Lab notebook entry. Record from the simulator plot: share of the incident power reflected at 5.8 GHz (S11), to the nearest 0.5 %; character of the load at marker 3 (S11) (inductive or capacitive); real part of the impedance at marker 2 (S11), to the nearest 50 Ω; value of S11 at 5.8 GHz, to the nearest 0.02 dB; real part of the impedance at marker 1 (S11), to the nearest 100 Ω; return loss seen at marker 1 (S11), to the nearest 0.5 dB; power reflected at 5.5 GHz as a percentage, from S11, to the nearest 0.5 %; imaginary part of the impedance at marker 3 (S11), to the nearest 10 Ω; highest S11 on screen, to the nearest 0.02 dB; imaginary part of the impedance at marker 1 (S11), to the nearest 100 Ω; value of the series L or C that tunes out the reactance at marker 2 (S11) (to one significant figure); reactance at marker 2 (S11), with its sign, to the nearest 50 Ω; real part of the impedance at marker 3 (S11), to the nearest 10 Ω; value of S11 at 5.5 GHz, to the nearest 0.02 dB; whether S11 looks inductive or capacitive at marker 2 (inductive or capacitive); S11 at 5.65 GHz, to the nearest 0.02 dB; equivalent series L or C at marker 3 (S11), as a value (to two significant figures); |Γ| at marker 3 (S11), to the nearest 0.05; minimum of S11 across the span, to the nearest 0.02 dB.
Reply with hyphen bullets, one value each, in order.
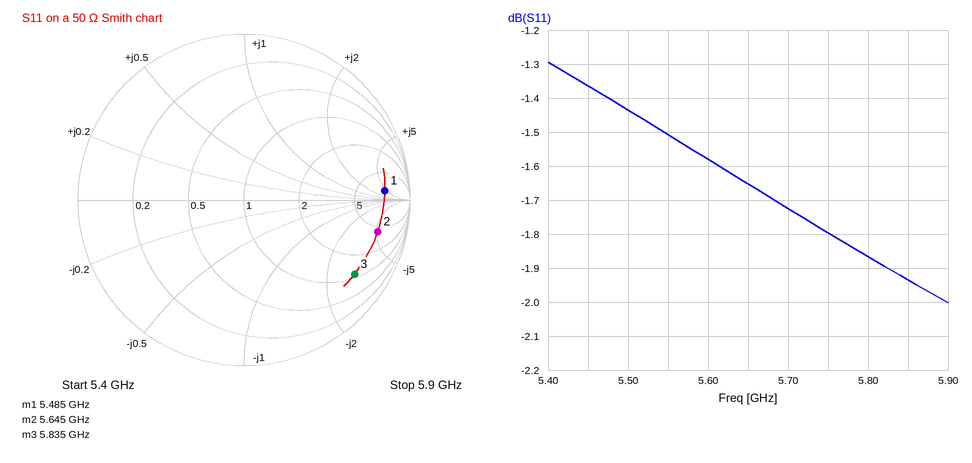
- 65.0 %
- capacitive
- 200 Ω
- -1.86 dB
- 500 Ω
- 1.5 dB
- 72.0 %
- -140 Ω
- -1.30 dB
- +200 Ω
- 7 nH
- -250 Ω
- 60 Ω
- -1.44 dB
- capacitive
- -1.66 dB
- 190 fF
- 0.80
- -2.00 dB
